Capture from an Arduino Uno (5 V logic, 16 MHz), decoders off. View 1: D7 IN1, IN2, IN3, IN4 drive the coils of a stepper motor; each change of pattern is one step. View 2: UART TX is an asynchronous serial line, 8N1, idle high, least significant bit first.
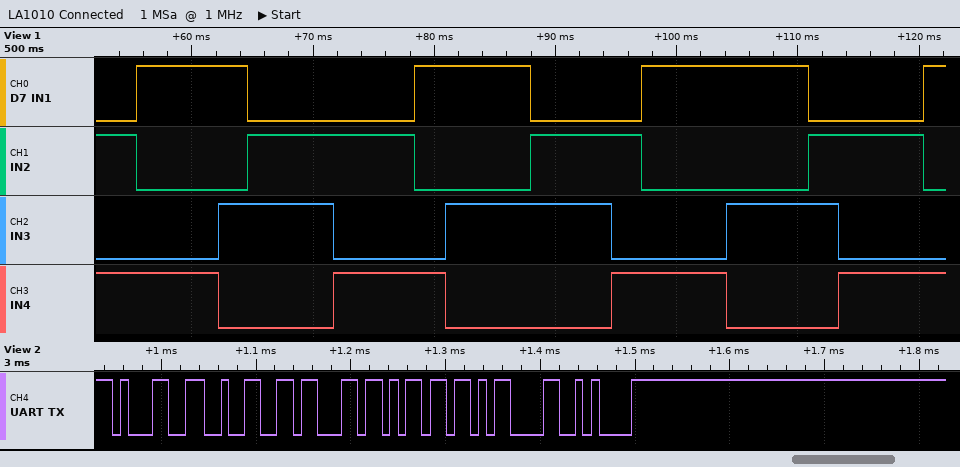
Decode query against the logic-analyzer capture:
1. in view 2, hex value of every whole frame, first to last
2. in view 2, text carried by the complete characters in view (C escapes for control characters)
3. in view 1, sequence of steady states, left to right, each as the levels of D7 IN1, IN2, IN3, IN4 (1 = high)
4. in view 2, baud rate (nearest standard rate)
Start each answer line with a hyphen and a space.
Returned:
- 0x31 0x32 0x63 0x6D 0x0D 0x0A
- "12cm\r\n"
- 0101 1001 1010 0110 0101 1001 1010 0110 0101 1001 1010 0110 0101 1001
- 115200 baud
